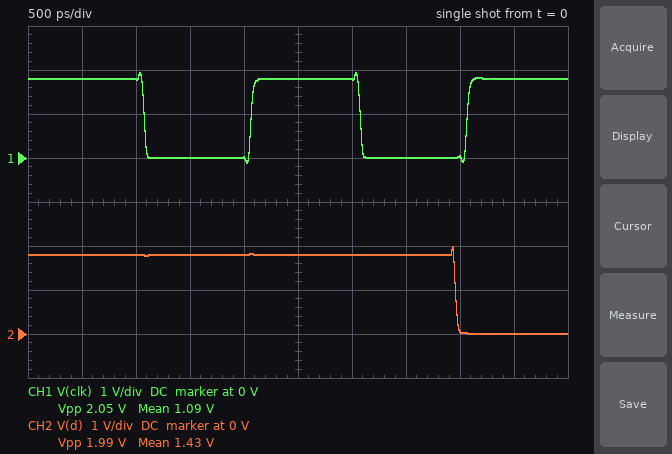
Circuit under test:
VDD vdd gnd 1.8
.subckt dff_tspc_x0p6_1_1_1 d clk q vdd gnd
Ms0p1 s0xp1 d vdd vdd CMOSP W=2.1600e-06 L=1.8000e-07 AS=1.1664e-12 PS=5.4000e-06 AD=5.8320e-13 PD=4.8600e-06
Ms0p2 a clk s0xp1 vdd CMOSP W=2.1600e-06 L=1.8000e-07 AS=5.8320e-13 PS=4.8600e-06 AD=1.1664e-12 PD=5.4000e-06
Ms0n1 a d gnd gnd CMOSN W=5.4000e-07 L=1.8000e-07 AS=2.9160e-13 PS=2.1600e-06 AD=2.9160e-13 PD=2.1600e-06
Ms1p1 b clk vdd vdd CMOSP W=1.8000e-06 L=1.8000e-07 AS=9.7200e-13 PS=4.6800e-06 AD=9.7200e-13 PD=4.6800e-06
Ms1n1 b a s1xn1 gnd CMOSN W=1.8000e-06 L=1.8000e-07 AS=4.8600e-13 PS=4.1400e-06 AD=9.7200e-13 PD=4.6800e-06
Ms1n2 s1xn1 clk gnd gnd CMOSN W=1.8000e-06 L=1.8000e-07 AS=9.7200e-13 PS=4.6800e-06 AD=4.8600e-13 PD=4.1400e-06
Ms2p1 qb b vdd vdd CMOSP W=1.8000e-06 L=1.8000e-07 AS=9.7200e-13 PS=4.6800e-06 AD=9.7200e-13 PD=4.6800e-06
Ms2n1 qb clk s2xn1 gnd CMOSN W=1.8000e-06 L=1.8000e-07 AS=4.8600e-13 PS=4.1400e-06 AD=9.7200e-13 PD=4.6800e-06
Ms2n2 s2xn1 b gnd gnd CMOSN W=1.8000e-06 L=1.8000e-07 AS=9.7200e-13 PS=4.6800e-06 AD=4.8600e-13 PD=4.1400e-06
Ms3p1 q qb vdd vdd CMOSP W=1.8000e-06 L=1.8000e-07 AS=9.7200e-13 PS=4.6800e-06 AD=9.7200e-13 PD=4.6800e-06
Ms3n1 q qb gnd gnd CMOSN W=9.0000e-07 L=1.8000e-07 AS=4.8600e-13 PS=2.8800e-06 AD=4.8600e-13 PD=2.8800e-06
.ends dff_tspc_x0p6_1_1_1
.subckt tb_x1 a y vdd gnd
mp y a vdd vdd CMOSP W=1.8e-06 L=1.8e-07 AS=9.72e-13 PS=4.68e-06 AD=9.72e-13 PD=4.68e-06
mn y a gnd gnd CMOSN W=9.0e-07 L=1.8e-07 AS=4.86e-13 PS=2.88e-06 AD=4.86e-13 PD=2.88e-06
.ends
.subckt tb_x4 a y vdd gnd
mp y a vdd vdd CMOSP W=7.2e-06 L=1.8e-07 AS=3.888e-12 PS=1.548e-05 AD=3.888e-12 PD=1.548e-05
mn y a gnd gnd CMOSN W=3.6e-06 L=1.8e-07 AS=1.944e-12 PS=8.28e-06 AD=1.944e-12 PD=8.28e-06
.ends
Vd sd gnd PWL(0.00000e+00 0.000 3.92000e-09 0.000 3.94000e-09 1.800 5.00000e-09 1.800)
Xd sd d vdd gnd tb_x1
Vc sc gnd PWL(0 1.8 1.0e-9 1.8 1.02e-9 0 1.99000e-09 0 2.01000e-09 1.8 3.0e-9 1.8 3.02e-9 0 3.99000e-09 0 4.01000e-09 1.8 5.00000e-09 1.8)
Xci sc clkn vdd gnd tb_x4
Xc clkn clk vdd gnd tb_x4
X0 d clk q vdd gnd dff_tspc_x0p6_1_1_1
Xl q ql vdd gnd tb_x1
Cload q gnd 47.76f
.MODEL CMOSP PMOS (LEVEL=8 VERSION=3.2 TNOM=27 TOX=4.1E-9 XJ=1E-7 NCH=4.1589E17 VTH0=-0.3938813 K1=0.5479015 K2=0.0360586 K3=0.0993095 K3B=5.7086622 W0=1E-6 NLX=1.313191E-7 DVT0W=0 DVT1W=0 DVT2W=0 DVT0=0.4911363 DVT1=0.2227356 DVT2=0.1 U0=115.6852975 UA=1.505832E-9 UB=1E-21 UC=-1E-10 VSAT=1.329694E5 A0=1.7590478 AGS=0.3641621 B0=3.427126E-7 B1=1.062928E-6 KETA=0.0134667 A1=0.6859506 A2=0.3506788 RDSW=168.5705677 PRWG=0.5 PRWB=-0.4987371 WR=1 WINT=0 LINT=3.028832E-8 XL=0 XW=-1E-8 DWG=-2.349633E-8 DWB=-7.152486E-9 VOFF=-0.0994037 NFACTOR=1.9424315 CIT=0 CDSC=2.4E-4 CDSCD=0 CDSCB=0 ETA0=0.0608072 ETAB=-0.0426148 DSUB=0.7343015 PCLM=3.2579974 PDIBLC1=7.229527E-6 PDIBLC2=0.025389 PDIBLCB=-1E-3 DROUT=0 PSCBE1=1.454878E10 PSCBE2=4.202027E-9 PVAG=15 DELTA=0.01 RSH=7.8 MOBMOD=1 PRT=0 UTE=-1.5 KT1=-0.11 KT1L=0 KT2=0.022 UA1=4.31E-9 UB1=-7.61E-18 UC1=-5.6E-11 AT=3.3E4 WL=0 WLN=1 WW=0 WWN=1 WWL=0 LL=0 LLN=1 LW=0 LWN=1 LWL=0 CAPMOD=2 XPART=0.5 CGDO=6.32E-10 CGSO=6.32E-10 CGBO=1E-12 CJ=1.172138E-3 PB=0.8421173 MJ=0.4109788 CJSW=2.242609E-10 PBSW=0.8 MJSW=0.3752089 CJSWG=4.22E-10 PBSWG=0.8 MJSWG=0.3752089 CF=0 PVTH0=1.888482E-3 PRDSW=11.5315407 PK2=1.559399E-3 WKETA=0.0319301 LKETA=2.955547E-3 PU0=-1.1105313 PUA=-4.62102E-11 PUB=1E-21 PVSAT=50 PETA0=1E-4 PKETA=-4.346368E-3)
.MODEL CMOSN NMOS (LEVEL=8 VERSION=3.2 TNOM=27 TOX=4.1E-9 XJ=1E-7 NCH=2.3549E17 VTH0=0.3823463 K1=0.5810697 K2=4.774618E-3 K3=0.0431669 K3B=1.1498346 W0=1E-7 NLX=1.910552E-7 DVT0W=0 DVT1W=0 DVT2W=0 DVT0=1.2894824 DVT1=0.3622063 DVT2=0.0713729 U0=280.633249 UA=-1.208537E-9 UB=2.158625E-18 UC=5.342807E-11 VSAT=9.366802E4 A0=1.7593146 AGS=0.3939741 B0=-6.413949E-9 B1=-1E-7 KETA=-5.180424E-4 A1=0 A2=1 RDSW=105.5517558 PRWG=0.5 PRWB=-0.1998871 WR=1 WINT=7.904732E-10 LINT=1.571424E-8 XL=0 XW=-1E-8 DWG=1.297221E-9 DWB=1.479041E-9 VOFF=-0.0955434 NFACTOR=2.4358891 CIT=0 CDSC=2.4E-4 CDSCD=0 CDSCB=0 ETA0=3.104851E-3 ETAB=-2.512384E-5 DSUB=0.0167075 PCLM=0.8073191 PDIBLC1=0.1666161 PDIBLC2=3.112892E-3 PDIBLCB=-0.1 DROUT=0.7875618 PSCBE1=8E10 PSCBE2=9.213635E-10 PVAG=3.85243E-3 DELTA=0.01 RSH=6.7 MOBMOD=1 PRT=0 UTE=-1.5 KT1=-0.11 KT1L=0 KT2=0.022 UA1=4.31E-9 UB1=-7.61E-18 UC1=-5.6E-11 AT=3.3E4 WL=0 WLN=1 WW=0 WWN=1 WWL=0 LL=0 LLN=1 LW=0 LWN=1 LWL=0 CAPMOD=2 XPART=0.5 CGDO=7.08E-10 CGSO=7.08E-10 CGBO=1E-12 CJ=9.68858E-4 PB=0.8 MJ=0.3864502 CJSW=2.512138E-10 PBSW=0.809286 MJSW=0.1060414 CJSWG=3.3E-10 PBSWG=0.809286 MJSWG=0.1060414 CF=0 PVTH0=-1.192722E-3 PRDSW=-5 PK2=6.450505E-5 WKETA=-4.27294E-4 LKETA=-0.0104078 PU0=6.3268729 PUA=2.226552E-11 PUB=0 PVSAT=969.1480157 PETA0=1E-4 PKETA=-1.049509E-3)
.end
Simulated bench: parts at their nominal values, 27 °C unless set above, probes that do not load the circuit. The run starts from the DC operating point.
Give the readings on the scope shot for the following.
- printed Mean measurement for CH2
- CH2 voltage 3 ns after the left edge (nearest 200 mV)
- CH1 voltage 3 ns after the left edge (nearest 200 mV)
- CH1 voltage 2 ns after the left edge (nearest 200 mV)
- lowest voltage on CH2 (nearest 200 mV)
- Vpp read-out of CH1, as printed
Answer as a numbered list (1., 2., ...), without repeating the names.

1. 1.43 V
2. 1.8 V
3. 1.8 V
4. 0 V
5. 0 V
6. 2.05 V
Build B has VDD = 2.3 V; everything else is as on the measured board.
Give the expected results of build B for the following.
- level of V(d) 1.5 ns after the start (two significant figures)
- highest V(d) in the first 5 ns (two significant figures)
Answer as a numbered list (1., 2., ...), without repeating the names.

1. 2.3 V
2. 2.5 V
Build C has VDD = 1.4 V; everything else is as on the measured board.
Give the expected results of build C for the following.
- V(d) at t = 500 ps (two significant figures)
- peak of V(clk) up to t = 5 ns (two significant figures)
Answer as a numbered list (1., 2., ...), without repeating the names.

1. 1.4 V
2. 1.5 V
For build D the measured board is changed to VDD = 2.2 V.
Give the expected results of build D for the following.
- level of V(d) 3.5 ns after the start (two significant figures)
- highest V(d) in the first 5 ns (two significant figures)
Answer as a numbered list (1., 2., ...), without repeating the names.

1. 2.2 V
2. 2.4 V
